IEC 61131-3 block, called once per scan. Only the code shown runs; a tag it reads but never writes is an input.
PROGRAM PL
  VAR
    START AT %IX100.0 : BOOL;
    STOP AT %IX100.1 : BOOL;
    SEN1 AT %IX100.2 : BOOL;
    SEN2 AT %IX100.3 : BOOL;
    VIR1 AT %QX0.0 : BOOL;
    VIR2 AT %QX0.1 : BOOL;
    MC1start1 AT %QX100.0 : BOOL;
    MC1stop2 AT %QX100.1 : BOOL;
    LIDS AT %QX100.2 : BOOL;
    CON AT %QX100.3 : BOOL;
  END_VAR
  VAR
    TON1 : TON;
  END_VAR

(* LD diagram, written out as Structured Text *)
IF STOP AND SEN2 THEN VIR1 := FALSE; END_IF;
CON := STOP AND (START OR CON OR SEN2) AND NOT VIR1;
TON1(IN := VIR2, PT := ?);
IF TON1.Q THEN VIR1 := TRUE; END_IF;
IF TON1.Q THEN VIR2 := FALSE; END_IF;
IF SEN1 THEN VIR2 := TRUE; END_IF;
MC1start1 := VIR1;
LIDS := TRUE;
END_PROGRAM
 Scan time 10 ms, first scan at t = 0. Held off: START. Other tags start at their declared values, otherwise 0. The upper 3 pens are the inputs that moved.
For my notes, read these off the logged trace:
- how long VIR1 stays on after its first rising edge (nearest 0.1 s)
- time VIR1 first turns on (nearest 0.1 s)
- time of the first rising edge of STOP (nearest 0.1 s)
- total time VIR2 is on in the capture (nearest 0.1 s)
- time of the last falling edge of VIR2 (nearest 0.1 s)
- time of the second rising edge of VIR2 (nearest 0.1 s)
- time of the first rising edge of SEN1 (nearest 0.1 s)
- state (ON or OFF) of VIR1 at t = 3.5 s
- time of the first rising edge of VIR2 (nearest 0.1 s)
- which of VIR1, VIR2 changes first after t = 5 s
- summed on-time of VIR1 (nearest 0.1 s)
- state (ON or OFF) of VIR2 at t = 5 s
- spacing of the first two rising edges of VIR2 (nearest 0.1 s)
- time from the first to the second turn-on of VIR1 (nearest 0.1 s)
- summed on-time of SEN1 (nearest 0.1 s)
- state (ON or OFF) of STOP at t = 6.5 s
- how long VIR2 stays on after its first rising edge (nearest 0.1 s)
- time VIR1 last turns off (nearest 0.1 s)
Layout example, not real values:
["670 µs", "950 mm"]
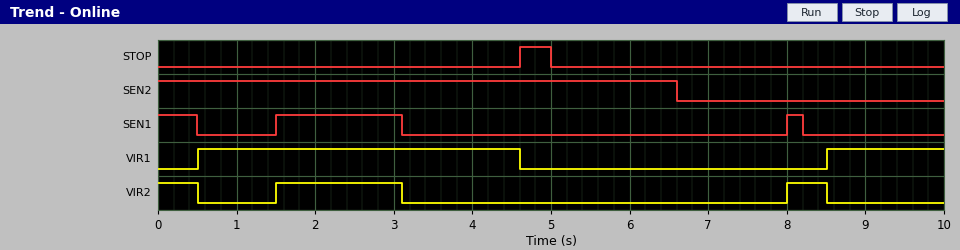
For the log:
["4.1 s", "0.5 s", "4.6 s", "2.6 s", "8.5 s", "8.0 s", "1.5 s", "ON", "1.5 s", "VIR2", "5.6 s", "OFF", "6.5 s", "8.0 s", "2.3 s", "OFF", "1.6 s", "4.6 s"]
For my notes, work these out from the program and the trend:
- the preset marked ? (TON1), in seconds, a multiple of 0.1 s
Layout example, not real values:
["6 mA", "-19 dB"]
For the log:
["0.5 s"]
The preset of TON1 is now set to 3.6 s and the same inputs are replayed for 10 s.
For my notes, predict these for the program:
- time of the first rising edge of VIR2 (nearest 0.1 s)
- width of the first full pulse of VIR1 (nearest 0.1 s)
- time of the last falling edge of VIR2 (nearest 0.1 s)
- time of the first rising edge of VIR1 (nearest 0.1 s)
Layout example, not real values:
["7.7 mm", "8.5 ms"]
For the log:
["8.0 s", "1.0 s", "3.6 s", "3.6 s"]
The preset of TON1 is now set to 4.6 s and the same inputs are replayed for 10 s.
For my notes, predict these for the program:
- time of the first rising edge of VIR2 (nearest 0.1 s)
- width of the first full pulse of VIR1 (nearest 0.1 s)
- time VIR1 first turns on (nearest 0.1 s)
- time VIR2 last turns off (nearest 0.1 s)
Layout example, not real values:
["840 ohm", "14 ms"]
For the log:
["8.0 s", "0.0 s", "4.6 s", "4.6 s"]
